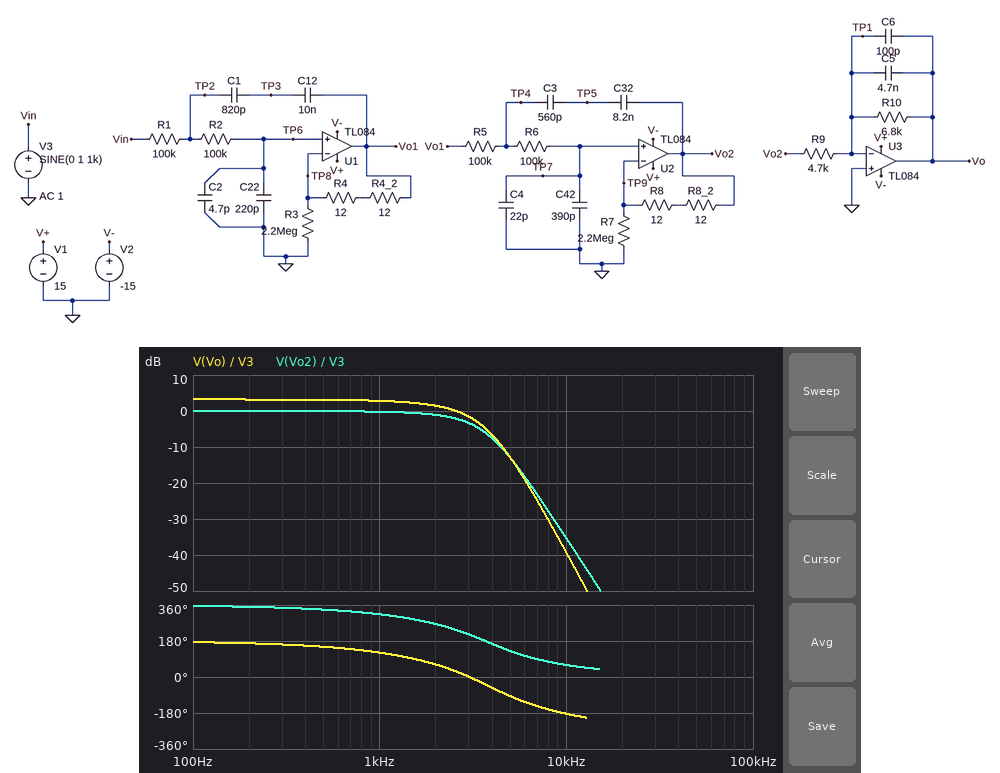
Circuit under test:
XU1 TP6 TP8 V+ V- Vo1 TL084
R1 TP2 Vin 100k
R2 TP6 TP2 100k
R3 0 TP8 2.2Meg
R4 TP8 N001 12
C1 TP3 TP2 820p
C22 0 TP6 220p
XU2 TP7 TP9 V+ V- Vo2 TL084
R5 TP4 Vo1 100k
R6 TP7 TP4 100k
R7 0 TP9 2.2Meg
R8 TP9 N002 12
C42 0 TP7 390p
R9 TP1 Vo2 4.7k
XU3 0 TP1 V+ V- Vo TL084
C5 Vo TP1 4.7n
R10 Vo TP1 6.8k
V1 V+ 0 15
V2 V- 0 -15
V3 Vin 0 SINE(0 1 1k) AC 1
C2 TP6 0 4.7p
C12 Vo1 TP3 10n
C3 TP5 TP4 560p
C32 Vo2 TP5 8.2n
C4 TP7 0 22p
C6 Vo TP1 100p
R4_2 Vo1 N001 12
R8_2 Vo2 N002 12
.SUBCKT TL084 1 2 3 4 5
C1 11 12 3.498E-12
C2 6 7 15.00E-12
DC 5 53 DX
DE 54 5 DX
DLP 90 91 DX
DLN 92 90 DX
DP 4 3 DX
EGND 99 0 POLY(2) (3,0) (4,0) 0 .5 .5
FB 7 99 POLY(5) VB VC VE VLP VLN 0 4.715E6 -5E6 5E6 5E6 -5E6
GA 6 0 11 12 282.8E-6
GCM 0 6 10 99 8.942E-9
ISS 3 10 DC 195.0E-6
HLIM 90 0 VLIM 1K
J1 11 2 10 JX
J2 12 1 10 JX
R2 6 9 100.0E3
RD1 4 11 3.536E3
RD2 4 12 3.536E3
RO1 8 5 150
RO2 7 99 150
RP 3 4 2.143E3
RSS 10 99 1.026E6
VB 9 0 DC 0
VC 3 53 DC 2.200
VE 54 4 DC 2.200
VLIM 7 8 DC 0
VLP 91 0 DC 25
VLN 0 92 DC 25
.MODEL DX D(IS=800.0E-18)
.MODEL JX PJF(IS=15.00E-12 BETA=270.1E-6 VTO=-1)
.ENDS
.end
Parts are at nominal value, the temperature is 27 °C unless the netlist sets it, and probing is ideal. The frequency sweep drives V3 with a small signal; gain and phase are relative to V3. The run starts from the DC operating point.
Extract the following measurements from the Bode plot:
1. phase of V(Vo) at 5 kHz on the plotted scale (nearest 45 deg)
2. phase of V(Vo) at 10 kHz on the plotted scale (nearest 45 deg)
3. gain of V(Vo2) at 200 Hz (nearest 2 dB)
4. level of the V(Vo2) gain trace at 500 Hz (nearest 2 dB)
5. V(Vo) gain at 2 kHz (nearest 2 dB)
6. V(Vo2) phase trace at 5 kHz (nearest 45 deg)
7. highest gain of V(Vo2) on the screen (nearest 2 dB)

-90 deg
-180 deg
0 dB
0 dB
2 dB
135 deg
0 dB
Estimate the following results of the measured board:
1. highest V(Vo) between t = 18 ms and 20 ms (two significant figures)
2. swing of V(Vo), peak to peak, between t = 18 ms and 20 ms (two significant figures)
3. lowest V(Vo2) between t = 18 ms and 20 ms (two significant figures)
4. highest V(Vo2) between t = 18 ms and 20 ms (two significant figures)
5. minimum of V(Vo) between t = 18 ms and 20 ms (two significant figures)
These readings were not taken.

1.4 V
2.8 V
-980 mV
980 mV
-1.4 V
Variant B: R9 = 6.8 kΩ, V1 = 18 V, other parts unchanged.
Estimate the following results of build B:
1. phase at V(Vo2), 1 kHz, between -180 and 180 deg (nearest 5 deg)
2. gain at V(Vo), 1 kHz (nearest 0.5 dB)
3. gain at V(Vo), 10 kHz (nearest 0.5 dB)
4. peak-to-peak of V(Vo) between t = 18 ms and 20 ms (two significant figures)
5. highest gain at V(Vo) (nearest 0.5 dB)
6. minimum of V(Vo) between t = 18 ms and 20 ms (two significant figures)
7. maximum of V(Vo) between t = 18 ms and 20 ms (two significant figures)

-45 deg
-0.5 dB
-42.5 dB
1.9 V
0 dB
-960 mV
960 mV
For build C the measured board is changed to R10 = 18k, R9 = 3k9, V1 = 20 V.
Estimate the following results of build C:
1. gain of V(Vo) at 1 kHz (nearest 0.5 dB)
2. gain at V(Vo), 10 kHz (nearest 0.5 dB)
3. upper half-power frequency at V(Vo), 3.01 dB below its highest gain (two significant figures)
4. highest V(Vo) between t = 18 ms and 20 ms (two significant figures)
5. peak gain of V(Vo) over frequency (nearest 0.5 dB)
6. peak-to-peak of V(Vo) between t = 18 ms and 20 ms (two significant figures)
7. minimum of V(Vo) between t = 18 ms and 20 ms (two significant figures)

12.0 dB
-37.0 dB
1.6 kHz
4.0 V
13.5 dB
7.9 V
-4.0 V
